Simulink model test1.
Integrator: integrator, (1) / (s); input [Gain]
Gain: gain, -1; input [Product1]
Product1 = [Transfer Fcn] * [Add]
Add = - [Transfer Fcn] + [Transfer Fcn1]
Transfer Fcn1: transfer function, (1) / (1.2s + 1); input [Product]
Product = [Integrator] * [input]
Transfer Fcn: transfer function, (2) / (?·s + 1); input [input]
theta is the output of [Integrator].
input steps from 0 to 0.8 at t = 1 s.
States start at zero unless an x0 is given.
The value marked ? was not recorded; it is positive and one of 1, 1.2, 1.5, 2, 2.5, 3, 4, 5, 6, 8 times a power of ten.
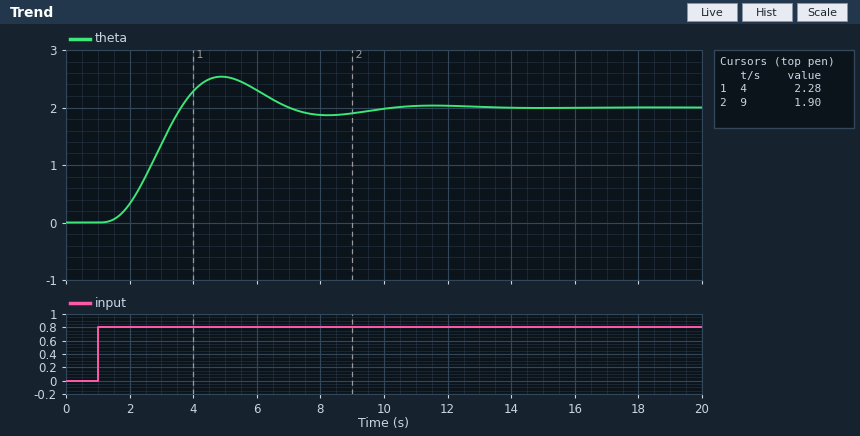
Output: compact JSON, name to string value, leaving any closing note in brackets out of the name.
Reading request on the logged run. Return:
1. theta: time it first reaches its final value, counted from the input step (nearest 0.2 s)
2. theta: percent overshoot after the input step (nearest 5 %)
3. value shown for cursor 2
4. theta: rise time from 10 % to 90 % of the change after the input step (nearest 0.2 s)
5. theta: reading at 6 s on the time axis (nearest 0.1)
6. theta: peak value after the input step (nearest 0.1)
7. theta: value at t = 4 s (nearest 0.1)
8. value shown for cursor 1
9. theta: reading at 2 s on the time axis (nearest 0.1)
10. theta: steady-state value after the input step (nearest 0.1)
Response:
{"theta: time it first reaches its final value, counted from the input step": "2.6 s", "theta: percent overshoot after the input step": "25 %", "value shown for cursor 2": "1.90", "theta: rise time from 10 % to 90 % of the change after the input step": "1.6 s", "theta: reading at 6 s on the time axis": "2.3", "theta: peak value after the input step": "2.5", "theta: value at t = 4 s": "2.3", "value shown for cursor 1": "2.28", "theta: reading at 2 s on the time axis": "0.3", "theta: steady-state value after the input step": "2.0"}
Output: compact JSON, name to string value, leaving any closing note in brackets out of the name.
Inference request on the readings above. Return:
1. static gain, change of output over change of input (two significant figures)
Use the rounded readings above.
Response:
{"static gain, change of output over change of input": "2.5"}
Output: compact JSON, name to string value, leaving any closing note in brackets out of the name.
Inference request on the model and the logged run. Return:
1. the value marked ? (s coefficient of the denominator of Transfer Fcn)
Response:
{"the value marked ?": "1.2"}
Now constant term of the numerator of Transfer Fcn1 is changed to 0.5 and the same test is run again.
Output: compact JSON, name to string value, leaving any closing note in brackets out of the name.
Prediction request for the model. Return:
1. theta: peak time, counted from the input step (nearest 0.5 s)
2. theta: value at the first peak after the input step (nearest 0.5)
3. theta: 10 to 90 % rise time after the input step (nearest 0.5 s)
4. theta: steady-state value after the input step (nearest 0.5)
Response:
{"theta: peak time, counted from the input step": "6.0 s", "theta: value at the first peak after the input step": "4.5", "theta: 10 to 90 % rise time after the input step": "2.5 s", "theta: steady-state value after the input step": "4.0"}
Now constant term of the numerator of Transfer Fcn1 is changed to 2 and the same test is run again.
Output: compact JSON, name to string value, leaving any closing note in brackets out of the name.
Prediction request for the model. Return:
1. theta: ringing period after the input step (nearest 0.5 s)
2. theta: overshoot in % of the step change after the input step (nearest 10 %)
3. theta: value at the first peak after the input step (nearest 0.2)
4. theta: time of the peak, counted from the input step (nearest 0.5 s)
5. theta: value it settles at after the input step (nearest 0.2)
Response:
{"theta: ringing period after the input step": "4.5 s", "theta: overshoot in % of the step change after the input step": "40 %", "theta: value at the first peak after the input step": "1.4", "theta: time of the peak, counted from the input step": "3.0 s", "theta: value it settles at after the input step": "1.0"}
